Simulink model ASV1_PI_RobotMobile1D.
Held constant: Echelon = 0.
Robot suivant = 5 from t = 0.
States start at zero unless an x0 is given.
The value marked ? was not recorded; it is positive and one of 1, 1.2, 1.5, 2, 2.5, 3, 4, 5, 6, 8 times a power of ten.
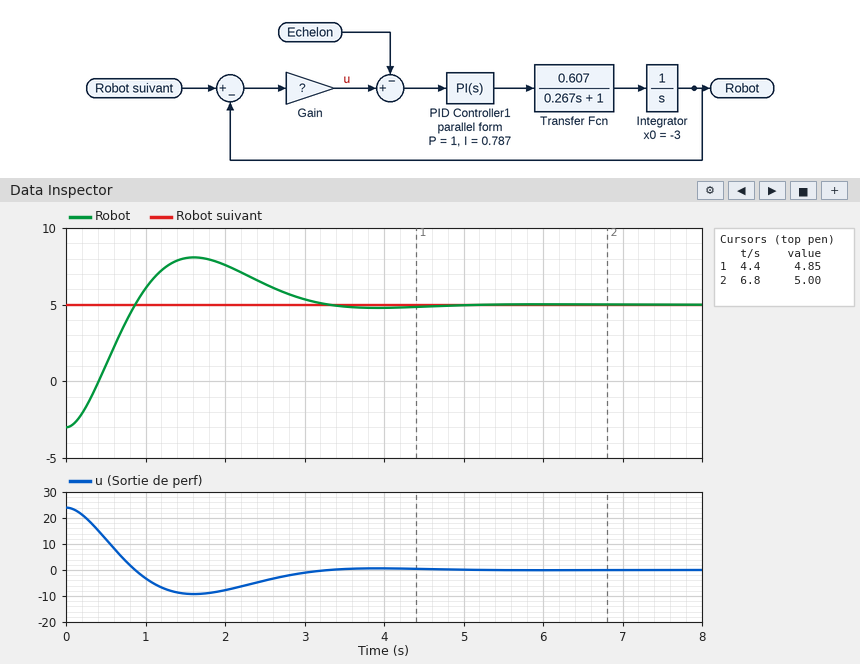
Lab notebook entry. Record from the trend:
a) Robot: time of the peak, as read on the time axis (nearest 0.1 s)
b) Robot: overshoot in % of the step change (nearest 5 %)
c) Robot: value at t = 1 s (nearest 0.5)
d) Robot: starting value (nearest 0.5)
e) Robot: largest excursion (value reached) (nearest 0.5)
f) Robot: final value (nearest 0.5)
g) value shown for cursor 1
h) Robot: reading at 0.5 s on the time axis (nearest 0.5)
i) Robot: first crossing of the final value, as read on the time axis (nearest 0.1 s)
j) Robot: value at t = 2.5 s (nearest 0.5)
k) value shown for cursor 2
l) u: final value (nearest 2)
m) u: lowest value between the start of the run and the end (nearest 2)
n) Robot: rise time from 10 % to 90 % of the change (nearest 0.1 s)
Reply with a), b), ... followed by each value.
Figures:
a) 1.6 s
b) 40 %
c) 6.0
d) -3.0
e) 8.0
f) 5.0
g) 4.85
h) 1.0
i) 0.9 s
j) 6.5
k) 5.00
l) 0
m) -10
n) 0.6 s
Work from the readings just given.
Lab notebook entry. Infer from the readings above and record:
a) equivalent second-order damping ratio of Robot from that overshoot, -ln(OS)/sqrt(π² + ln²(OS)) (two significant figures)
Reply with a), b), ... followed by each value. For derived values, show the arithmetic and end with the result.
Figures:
a) ln(0.4) = -0.916; 0.916 / sqrt(9.870 + 0.840) = 0.28
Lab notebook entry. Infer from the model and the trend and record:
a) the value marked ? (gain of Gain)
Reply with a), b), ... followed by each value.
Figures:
a) 3
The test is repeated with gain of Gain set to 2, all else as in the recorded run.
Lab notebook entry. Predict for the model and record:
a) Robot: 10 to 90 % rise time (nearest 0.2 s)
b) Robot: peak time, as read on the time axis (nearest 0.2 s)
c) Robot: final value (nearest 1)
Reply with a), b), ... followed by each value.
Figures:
a) 0.8 s
b) 2.2 s
c) 5
